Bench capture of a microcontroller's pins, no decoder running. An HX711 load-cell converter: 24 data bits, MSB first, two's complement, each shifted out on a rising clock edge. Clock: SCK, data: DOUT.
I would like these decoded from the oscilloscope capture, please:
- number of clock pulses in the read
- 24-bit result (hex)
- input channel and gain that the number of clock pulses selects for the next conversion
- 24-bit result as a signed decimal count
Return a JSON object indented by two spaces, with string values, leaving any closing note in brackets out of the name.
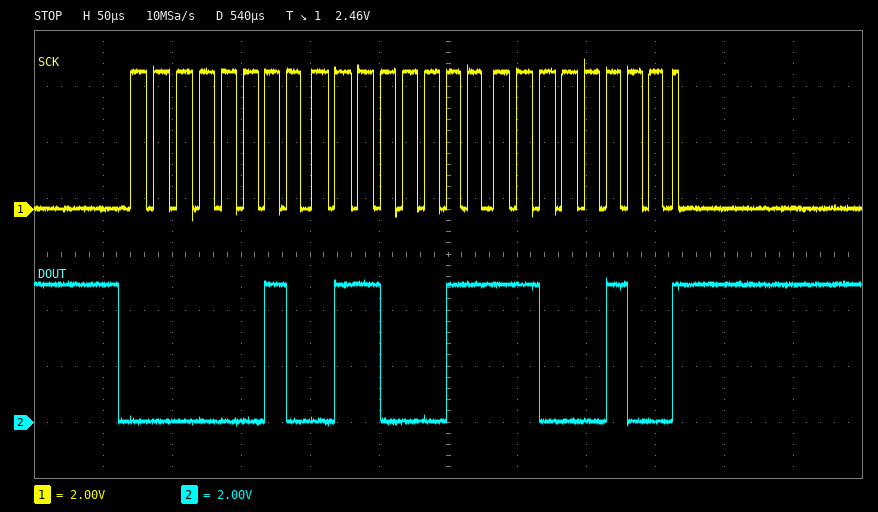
{
  "number of clock pulses in the read": "25",
  "24-bit result": "0x0263C4",
  "input channel and gain that the number of clock pulses selects for the next conversion": "channel A, gain 128",
  "24-bit result as a signed decimal count": "156612"
}
